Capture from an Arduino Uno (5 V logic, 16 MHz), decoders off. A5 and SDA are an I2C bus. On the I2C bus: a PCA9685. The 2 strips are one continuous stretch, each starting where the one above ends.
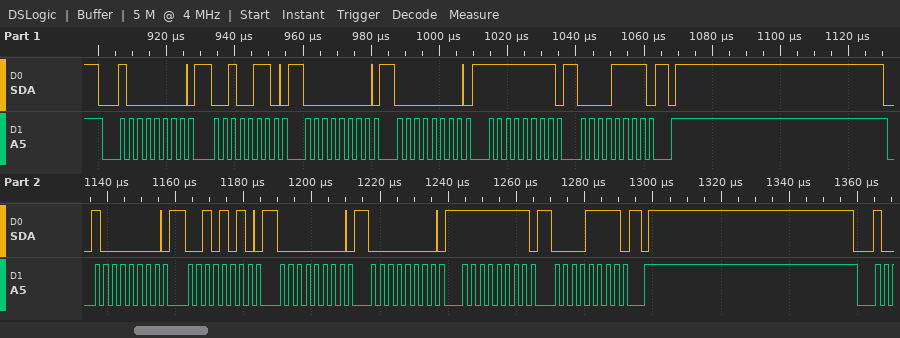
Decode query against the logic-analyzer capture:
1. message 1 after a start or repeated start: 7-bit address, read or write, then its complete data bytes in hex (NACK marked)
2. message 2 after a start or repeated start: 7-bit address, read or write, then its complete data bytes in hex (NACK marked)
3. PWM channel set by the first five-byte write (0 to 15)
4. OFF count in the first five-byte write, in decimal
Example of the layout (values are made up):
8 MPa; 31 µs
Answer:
0x40 write: 26 00 00 FF 0F; 0x40 write: 2A 00 00 FF 0F; 8; 4095
